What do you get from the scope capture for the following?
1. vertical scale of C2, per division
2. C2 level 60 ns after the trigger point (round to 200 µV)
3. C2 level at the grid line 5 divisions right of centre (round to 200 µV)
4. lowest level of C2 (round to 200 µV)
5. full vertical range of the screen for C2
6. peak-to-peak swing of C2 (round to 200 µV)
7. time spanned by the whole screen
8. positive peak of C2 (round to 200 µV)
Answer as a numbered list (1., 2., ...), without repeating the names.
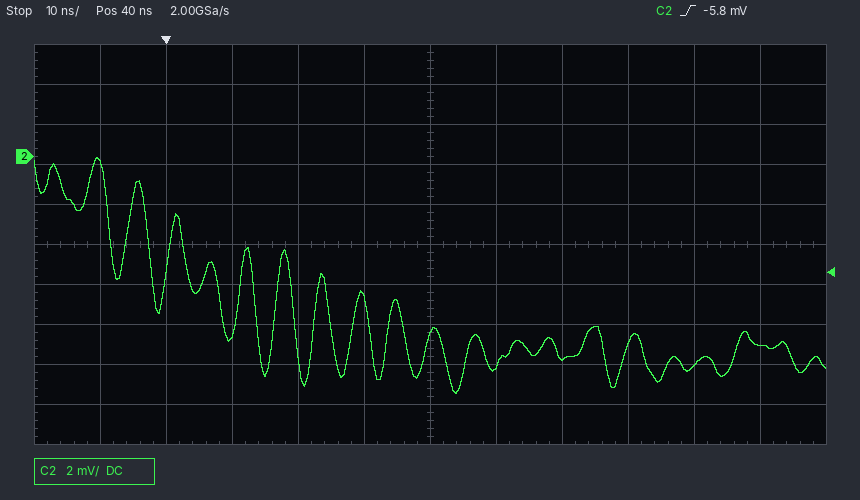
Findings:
1. 2 mV
2. -10.2 mV
3. -9.4 mV
4. -11.8 mV
5. 20 mV
6. 11.8 mV
7. 120 ns
8. 0.0 mV
